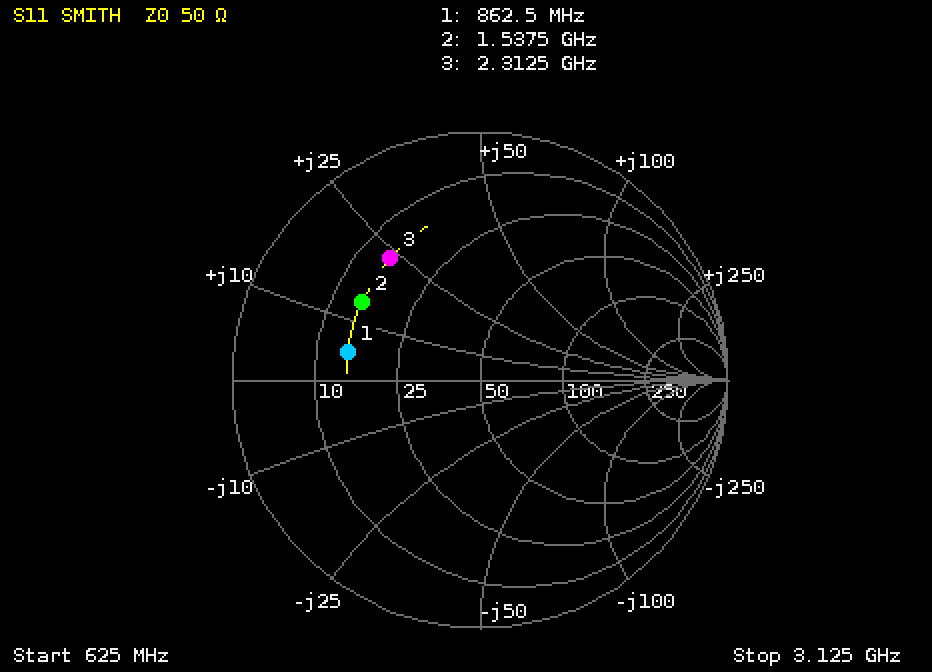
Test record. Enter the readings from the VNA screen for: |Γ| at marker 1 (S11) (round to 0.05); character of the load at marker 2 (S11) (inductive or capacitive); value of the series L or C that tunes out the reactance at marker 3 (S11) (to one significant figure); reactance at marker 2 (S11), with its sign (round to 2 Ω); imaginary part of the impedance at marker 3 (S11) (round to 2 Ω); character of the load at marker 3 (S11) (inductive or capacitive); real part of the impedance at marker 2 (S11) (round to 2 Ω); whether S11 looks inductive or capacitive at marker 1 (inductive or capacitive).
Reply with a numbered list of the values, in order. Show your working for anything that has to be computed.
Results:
1. 0.55
2. inductive
3. C = 1/(2π × 2.3125 GHz × 24 Ω) ≈ 3 pF
4. +14 Ω
5. +24 Ω
6. inductive
7. 14 Ω
8. inductive
